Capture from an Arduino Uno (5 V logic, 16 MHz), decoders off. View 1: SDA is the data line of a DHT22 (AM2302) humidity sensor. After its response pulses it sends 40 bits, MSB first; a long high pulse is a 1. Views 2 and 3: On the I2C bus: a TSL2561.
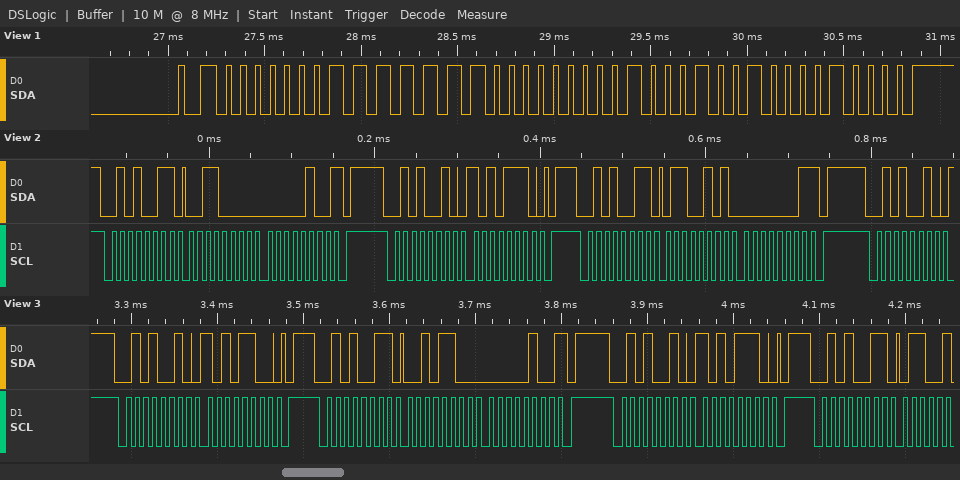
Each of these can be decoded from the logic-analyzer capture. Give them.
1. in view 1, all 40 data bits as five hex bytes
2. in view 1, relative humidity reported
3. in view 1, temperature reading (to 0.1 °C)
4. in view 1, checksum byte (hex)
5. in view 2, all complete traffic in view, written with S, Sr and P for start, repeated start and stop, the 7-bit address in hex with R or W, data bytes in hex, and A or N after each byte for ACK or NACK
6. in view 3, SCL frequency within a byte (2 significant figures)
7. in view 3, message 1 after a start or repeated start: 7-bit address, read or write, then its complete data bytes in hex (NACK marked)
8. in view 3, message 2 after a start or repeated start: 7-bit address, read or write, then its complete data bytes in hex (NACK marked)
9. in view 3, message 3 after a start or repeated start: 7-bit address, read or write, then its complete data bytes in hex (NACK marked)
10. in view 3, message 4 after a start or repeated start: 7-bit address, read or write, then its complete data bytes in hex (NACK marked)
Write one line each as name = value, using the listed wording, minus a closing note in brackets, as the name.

in view 1, all 40 data bits as five hex bytes = 01 FC 01 12 10
in view 1, relative humidity reported = 50.8 %
in view 1, temperature reading = 27.4 °C
in view 1, checksum byte = 0x10
in view 2, all complete traffic in view, written with S, Sr and P for start, repeated start and stop, the 7-bit address in hex with R or W, data bytes in hex, and A or N after each byte for ACK or NACK = S 29R A 30 A 04 N P S 29W A AE A P S 29R A 65 A 01 N P S 29W A
in view 3, SCL frequency within a byte = 100 kHz
in view 3, message 1 after a start or repeated start: 7-bit address, read or write, then its complete data bytes in hex = 0x29 write: AC
in view 3, message 2 after a start or repeated start: 7-bit address, read or write, then its complete data bytes in hex = 0x29 read: 2C 04 NACK
in view 3, message 3 after a start or repeated start: 7-bit address, read or write, then its complete data bytes in hex = 0x29 write: AE
in view 3, message 4 after a start or repeated start: 7-bit address, read or write, then its complete data bytes in hex = 0x29 read
